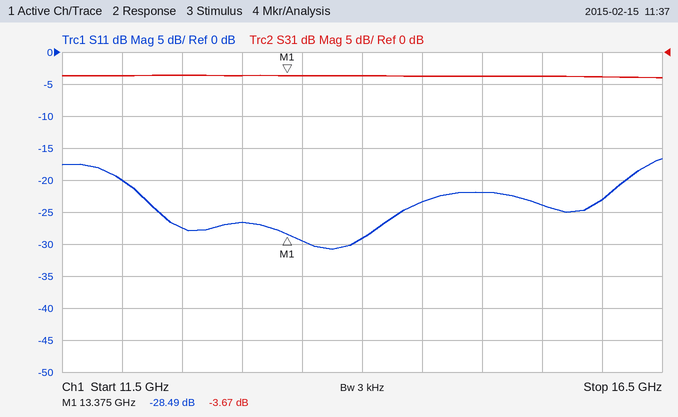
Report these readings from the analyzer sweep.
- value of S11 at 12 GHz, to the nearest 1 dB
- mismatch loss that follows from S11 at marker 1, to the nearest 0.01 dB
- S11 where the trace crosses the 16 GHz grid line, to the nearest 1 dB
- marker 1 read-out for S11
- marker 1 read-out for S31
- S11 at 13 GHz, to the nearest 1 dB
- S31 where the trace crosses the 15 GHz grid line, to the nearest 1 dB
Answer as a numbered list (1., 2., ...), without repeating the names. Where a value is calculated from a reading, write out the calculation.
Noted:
1. -20 dB
2. −10 log10(1 − 10^(-28.49/10)) ≈ 0.01 dB
3. -23 dB
4. -28.49 dB
5. -3.67 dB
6. -27 dB
7. -4 dB
